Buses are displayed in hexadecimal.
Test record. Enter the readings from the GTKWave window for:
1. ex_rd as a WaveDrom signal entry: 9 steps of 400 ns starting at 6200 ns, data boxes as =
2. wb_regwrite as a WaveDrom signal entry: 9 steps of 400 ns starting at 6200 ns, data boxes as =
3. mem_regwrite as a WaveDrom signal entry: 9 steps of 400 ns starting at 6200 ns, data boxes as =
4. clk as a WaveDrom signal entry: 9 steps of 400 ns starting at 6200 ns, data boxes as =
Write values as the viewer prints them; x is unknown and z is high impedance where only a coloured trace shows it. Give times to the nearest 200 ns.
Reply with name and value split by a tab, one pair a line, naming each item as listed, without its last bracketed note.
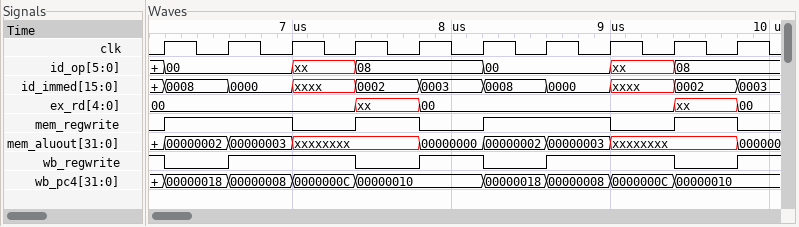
ex_rd as a WaveDrom signal entry: 9 steps of 400 ns starting at 6200 ns, data boxes as =	{name: 'ex_rd', wave: '=..x=...x', data: '00 00'}
wb_regwrite as a WaveDrom signal entry: 9 steps of 400 ns starting at 6200 ns, data boxes as =	{name: 'wb_regwrite', wave: '01.0101.0'}
mem_regwrite as a WaveDrom signal entry: 9 steps of 400 ns starting at 6200 ns, data boxes as =	{name: 'mem_regwrite', wave: '1.0101.01'}
clk as a WaveDrom signal entry: 9 steps of 400 ns starting at 6200 ns, data boxes as =	{name: 'clk', wave: 'p........'}
